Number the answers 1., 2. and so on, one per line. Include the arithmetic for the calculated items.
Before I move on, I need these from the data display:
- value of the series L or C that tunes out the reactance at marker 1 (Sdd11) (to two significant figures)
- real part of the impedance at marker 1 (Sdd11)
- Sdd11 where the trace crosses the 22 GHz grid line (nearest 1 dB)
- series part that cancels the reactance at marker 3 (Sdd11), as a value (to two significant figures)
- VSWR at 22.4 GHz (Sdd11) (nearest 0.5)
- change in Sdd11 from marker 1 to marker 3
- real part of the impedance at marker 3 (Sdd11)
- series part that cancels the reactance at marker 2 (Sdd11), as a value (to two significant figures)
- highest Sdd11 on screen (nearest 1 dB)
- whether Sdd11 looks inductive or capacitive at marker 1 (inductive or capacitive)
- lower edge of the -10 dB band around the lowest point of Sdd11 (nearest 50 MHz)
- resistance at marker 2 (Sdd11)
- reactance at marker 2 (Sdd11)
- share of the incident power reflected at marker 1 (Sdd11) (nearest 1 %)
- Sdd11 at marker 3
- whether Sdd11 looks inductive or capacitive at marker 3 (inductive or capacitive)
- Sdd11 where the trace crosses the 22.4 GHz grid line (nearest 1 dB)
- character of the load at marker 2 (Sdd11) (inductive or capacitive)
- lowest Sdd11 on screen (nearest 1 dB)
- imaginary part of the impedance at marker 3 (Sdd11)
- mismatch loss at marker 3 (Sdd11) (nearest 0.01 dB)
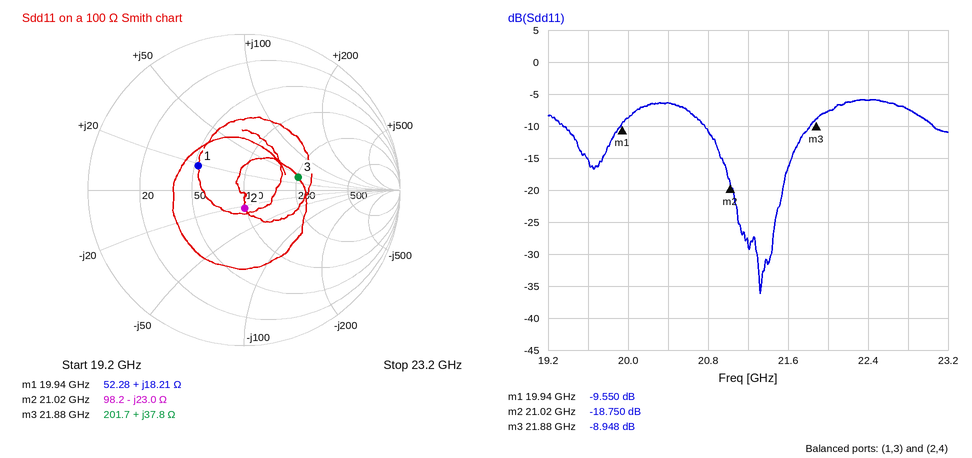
1. C = 1/(2π × 19.94 GHz × 18.21 Ω) ≈ 438 fF, so 440 fF to two significant figures
2. 52.28 Ω
3. -8 dB
4. C = 1/(2π × 21.88 GHz × 37.8 Ω) ≈ 192 fF, so 190 fF to two significant figures
5. |Γ| = 10^(-6/20) = 0.5012; VSWR = (1 + 0.5012)/(1 − 0.5012) ≈ 3.0
6. -8.948 − (-9.55) = 0.602 dB
7. 201.7 Ω
8. L = 23 Ω/(2π × 21.02 GHz) ≈ 174 pH, so 170 pH to two significant figures
9. -6 dB
10. inductive
11. 20.75 GHz
12. 98.2 Ω
13. -23.0 Ω
14. 10^(-9.55/10) ≈ 11 %
15. -8.948 dB
16. inductive
17. -6 dB
18. capacitive
19. -36 dB
20. +37.8 Ω
21. −10 log10(1 − 10^(-8.948/10)) ≈ 0.59 dB
